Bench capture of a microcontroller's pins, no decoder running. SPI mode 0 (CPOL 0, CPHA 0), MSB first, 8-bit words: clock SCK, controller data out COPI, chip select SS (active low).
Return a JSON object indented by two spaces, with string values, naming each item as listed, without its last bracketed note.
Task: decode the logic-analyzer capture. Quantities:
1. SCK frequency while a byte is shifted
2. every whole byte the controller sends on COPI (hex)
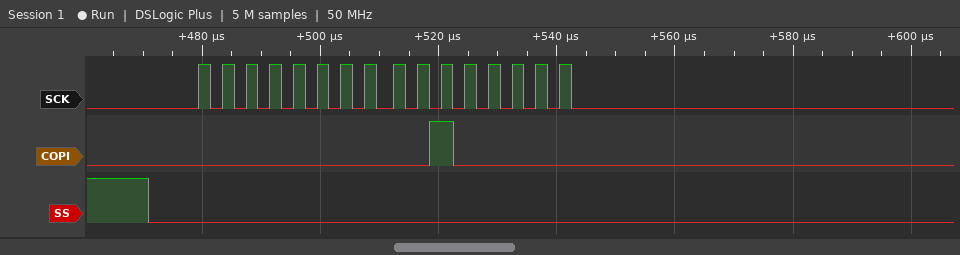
{
  "SCK frequency while a byte is shifted": "250 kHz",
  "every whole byte the controller sends on COPI": "00 20"
}
